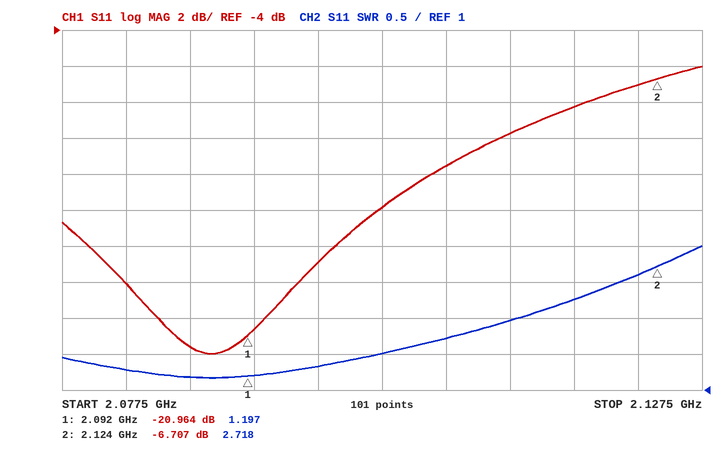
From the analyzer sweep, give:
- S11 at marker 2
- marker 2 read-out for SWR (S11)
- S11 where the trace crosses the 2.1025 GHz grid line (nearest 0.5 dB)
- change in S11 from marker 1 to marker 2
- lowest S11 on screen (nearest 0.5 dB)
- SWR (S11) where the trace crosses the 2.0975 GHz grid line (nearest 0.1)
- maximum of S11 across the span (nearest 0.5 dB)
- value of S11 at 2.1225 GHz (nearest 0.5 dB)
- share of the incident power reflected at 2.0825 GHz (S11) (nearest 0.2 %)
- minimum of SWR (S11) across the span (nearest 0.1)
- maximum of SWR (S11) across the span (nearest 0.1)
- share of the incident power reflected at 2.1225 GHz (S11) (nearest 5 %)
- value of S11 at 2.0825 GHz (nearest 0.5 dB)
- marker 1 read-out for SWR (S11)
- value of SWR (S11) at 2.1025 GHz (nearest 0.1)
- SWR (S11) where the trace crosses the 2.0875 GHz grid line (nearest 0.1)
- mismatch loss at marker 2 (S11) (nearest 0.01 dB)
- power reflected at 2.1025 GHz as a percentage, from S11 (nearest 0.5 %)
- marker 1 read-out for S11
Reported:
-6.707 dB
2.718
-14.0 dB
14.257 dB
-22.0 dB
1.3
-6.0 dB
-7.0 dB
1.6 %
1.2
3.0
20 %
-18.0 dB
1.197
1.5
1.2
1.04 dB
4.0 %
-20.964 dB
